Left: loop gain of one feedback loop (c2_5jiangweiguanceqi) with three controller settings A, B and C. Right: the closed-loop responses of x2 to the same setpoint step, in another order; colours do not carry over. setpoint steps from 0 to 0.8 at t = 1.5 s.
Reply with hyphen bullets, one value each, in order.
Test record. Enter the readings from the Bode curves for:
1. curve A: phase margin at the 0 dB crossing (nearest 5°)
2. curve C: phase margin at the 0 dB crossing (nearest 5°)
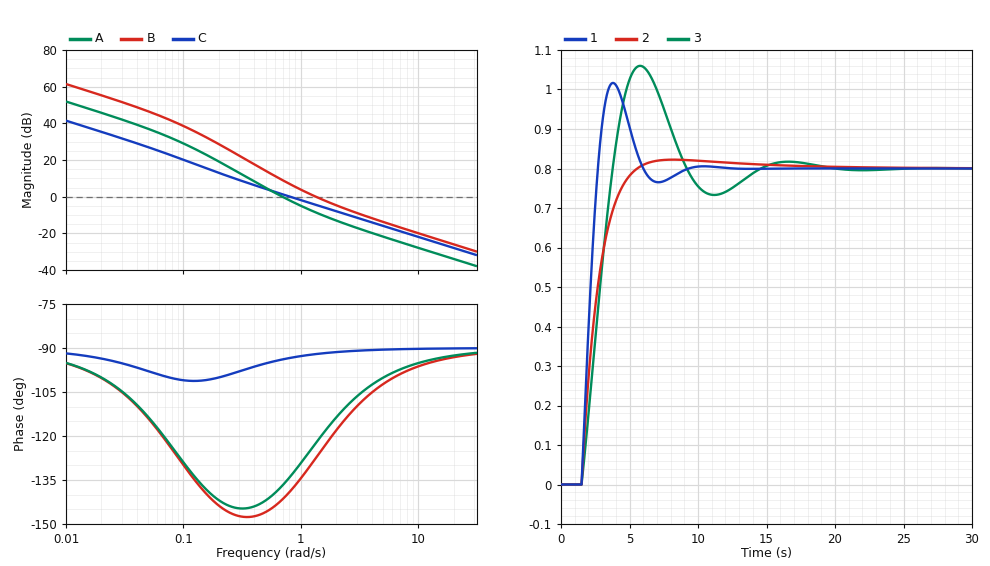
- 45°
- 85°
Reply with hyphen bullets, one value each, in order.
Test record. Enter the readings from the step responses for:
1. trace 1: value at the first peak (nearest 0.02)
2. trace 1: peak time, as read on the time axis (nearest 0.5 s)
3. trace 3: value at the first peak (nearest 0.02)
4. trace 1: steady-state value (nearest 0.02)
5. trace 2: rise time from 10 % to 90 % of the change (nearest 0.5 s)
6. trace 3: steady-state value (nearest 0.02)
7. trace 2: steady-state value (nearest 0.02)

- 1.02
- 4.0 s
- 1.06
- 0.80
- 2.5 s
- 0.80
- 0.80
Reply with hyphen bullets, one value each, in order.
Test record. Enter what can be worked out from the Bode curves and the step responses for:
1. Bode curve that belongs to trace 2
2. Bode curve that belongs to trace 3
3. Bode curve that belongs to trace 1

- C
- A
- B
